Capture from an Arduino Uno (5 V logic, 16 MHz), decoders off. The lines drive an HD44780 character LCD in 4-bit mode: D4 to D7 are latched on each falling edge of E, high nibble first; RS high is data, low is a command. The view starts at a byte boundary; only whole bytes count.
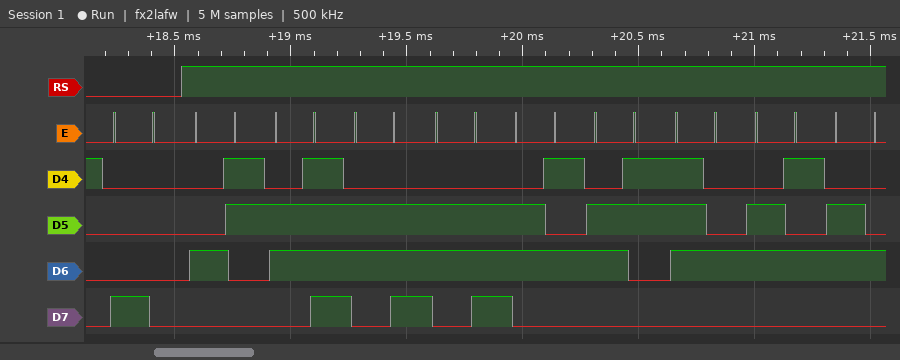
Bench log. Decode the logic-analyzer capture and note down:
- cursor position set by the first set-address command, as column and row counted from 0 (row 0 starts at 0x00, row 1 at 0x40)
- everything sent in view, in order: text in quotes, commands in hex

column 0, row 0
0x80 "Connected"
